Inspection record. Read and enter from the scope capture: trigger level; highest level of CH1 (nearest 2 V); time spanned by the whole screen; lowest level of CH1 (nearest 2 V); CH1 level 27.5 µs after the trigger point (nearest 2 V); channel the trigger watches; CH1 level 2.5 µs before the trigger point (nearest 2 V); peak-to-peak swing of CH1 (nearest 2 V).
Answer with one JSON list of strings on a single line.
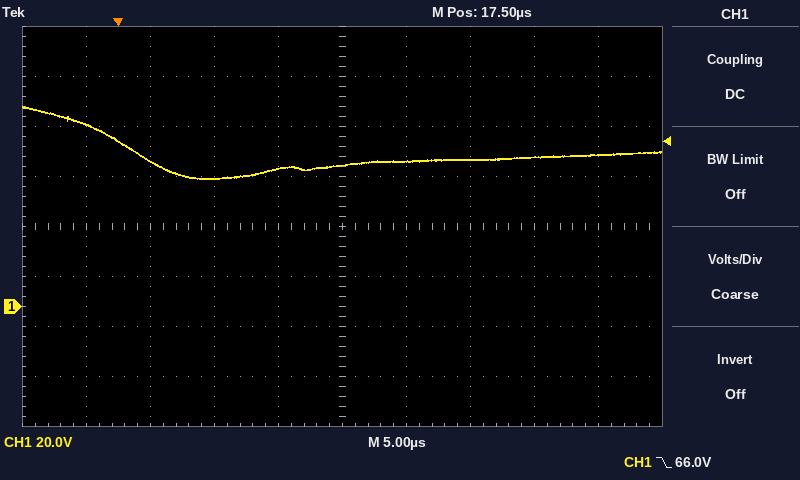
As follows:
["66.0 V", "80 V", "50 µs", "50 V", "58 V", "CH1", "72 V", "30 V"]
